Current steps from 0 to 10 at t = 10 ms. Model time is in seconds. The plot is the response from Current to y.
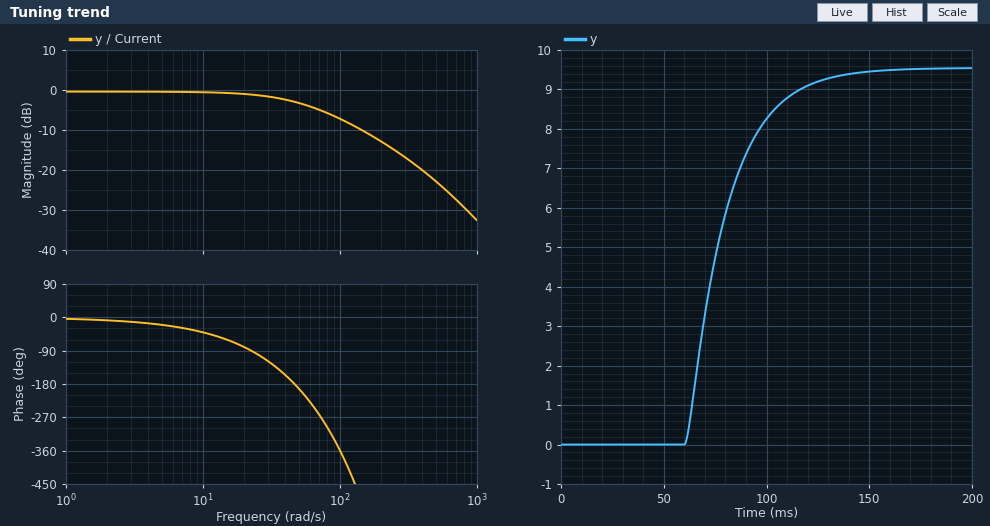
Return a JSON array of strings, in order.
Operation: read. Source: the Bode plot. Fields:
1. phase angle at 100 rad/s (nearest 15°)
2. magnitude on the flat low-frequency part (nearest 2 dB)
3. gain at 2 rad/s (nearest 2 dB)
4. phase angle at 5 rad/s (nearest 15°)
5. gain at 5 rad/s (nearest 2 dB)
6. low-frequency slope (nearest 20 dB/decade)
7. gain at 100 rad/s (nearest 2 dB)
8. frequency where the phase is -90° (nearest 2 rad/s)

["-360°", "0 dB", "0 dB", "-15°", "0 dB", "0 dB/decade", "-8 dB", "22 rad/s"]
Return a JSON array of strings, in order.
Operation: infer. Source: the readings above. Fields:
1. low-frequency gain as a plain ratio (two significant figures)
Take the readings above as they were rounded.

["1.0"]
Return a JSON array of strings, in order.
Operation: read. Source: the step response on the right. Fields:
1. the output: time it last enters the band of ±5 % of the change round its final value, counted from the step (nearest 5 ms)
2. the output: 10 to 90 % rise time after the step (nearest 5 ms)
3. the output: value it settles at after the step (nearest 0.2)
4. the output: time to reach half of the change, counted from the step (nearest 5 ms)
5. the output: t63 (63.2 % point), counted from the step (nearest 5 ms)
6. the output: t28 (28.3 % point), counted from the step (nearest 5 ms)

["110 ms", "40 ms", "9.6", "65 ms", "70 ms", "60 ms"]
